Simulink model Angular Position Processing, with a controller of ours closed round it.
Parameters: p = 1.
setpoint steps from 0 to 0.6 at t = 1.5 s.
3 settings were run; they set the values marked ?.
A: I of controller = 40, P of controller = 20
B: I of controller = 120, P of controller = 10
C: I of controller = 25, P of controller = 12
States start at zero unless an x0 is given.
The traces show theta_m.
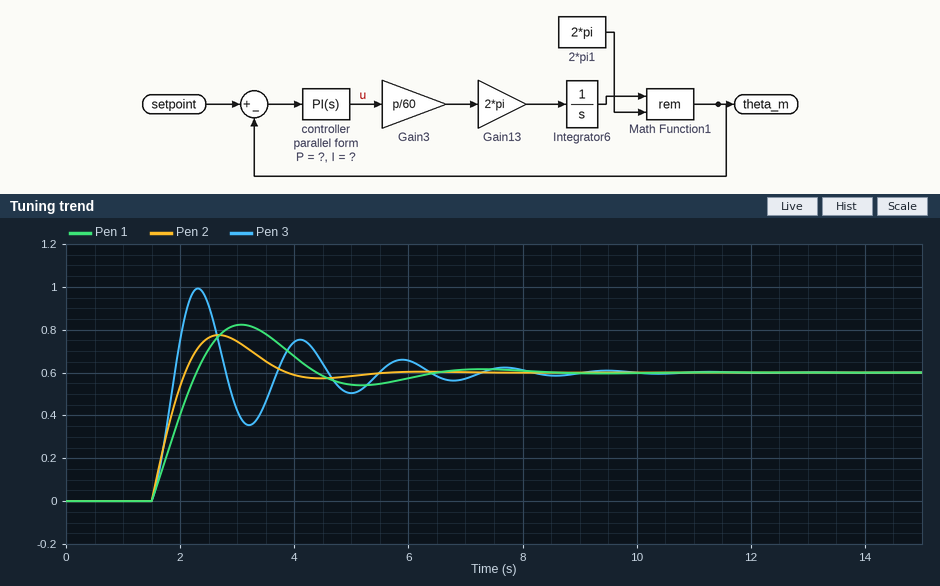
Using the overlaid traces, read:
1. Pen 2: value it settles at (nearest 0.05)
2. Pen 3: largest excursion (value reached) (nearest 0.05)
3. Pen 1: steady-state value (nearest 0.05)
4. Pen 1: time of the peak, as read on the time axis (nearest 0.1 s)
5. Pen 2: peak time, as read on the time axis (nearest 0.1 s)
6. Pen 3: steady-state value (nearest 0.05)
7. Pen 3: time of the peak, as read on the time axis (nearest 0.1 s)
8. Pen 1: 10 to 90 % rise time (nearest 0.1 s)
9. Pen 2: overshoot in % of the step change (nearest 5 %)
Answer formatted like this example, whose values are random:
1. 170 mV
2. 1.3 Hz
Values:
1. 0.60
2. 1.00
3. 0.60
4. 3.1 s
5. 2.7 s
6. 0.60
7. 2.3 s
8. 0.6 s
9. 30 %
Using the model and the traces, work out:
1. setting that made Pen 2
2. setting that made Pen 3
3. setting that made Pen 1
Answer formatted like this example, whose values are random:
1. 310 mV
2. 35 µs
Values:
1. A
2. B
3. C
